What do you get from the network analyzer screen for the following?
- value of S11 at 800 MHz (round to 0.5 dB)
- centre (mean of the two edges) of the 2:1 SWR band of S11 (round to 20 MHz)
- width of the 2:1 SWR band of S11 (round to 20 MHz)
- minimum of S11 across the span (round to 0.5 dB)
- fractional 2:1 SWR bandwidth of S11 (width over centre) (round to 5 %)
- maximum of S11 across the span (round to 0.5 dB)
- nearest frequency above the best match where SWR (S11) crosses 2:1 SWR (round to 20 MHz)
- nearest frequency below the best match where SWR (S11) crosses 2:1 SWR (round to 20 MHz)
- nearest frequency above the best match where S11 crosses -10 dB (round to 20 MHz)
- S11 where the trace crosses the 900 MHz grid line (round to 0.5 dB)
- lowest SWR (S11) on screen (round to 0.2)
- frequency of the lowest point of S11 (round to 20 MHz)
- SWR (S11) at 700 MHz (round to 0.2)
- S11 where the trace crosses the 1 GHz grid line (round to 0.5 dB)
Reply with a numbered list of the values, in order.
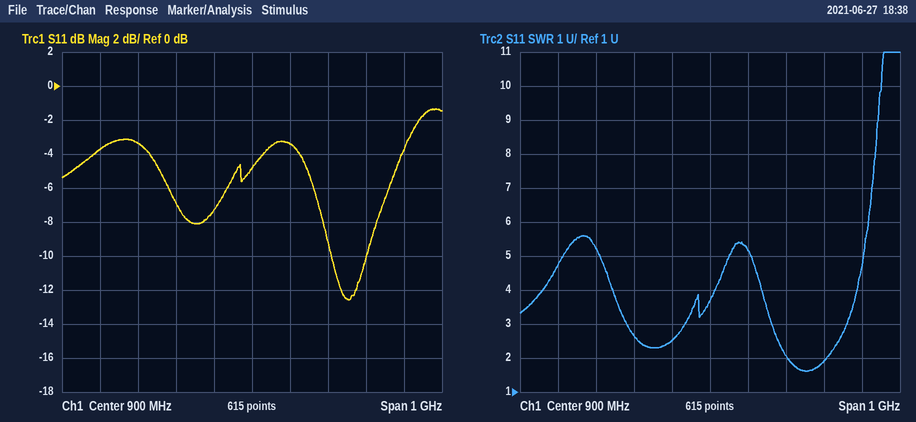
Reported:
1. -7.5 dB
2. 1.16 GHz
3. 100 MHz
4. -12.5 dB
5. 10 %
6. -1.5 dB
7. 1.20 GHz
8. 1.10 GHz
9. 1.20 GHz
10. -5.0 dB
11. 1.6
12. 1.16 GHz
13. 2.6
14. -3.5 dB
